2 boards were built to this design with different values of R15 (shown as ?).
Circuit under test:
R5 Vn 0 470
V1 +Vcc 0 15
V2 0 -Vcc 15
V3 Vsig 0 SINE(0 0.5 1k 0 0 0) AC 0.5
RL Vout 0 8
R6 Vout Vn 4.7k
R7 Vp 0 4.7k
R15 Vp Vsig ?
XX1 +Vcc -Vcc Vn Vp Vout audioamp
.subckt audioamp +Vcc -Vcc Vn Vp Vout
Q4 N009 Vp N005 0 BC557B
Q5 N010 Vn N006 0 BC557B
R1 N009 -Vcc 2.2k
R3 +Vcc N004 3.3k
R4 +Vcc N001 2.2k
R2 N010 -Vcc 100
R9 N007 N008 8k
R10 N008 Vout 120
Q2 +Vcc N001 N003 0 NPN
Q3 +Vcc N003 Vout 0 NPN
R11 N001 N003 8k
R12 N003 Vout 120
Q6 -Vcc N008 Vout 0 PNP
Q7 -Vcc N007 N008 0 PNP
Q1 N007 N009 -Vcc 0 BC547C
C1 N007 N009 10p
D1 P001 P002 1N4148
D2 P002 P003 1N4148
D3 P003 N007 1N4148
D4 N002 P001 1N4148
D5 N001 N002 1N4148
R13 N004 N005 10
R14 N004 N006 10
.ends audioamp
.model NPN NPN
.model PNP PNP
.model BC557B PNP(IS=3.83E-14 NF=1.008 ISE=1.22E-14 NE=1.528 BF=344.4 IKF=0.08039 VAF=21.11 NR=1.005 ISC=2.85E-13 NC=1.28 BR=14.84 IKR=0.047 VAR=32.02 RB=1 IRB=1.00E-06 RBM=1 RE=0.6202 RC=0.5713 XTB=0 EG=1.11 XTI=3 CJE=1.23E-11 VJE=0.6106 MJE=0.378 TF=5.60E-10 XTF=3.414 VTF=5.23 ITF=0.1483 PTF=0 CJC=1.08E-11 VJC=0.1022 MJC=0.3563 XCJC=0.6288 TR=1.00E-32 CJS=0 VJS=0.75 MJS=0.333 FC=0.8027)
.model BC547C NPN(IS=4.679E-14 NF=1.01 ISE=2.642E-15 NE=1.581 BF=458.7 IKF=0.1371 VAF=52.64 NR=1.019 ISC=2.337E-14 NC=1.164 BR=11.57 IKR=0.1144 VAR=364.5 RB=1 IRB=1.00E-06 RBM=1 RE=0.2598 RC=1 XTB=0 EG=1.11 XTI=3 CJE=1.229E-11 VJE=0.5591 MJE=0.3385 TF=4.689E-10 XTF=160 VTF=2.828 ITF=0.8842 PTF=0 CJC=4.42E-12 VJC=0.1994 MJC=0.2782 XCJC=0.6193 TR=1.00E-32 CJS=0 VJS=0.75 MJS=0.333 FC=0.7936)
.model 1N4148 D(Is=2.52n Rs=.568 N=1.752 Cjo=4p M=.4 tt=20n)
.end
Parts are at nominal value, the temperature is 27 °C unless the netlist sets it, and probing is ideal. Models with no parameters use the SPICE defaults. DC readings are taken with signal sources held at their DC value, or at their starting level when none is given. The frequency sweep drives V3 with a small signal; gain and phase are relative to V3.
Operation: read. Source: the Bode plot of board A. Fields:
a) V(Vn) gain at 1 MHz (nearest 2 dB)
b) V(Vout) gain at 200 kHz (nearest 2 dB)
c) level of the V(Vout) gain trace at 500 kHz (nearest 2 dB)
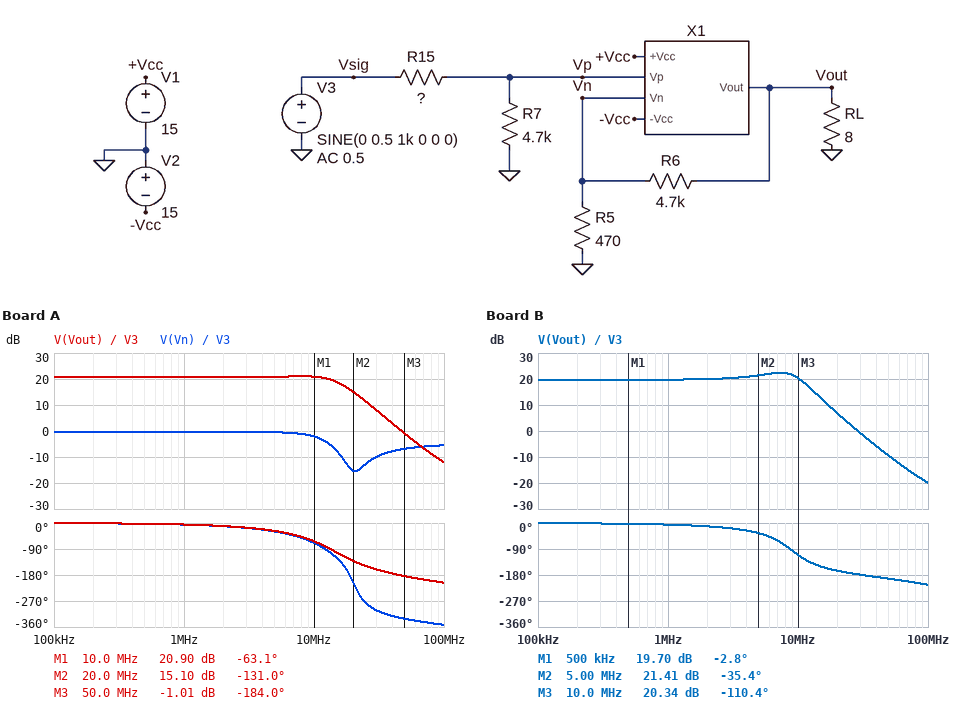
0 dB
20 dB
20 dB
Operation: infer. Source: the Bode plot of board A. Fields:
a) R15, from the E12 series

150 Ω
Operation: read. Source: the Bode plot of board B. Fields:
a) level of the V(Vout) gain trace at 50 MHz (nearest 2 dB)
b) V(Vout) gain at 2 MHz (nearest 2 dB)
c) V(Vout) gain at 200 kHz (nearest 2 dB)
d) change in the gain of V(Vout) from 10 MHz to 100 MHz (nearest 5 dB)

-10 dB
20 dB
20 dB
-40 dB
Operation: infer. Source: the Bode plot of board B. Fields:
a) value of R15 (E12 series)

680 Ω
